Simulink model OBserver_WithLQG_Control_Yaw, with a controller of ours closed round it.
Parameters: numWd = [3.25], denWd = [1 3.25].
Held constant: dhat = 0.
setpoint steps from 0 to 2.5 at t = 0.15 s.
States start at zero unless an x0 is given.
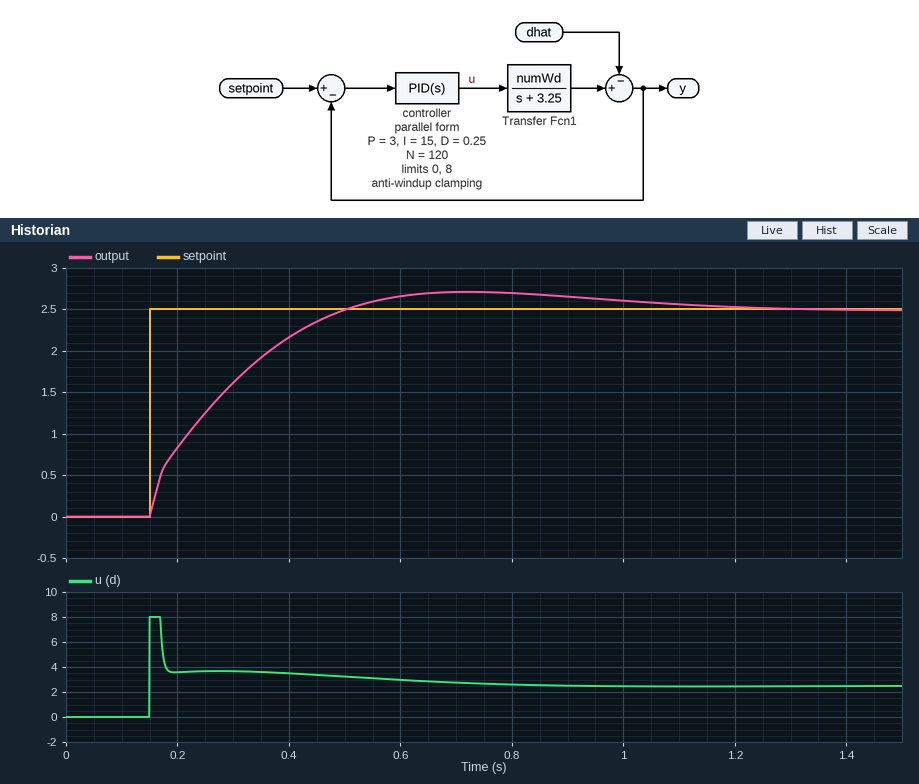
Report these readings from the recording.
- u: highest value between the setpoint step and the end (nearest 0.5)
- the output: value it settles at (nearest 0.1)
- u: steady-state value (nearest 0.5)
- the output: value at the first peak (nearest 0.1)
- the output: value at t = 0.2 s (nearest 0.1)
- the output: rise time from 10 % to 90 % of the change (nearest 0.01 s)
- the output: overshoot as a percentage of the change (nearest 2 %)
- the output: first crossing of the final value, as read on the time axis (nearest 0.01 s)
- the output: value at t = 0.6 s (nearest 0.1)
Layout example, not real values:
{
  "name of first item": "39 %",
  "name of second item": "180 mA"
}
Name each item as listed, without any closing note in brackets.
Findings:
{
  "u: highest value between the setpoint step and the end": "8.0",
  "the output: value it settles at": "2.5",
  "u: steady-state value": "2.5",
  "the output: value at the first peak": "2.7",
  "the output: value at t = 0.2 s": "0.8",
  "the output: rise time from 10 % to 90 % of the change": "0.26 s",
  "the output: overshoot as a percentage of the change": "8 %",
  "the output: first crossing of the final value, as read on the time axis": "0.50 s",
  "the output: value at t = 0.6 s": "2.7"
}
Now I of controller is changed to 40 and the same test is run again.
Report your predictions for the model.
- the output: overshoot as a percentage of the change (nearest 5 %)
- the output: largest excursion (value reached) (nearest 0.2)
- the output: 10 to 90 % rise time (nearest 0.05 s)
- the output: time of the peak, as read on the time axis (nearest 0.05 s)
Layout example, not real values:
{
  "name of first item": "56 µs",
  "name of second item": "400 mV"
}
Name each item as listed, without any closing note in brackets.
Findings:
{
  "the output: overshoot as a percentage of the change": "20 %",
  "the output: largest excursion (value reached)": "3.0",
  "the output: 10 to 90 % rise time": "0.15 s",
  "the output: time of the peak, as read on the time axis": "0.50 s"
}
